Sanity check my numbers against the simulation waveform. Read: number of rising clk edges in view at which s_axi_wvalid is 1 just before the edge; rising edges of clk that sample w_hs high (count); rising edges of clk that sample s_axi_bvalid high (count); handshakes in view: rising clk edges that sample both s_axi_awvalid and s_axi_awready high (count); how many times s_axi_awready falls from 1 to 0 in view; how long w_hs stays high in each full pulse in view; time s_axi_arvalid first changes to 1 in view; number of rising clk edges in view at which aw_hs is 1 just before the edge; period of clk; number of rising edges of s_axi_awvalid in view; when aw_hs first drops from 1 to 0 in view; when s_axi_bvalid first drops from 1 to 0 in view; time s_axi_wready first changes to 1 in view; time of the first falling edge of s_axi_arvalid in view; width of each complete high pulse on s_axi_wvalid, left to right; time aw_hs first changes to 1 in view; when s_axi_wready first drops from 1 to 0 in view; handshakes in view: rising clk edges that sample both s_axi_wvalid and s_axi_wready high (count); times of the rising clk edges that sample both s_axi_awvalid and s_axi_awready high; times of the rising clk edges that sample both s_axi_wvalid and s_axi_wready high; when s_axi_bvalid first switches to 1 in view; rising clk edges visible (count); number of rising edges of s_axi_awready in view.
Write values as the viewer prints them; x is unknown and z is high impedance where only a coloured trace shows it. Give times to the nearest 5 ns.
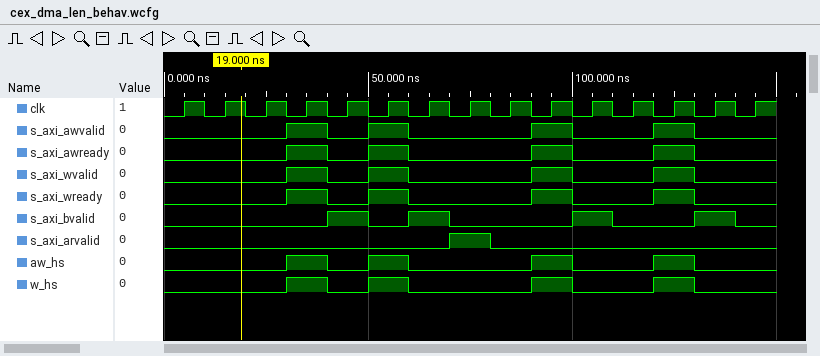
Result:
4
4
4
4
4
10 ns, 10 ns, 10 ns, 10 ns
70 ns
4
10 ns
4
40 ns
50 ns
30 ns
80 ns
10 ns, 10 ns, 10 ns, 10 ns
30 ns
40 ns
4
35 ns, 55 ns, 95 ns, 125 ns
35 ns, 55 ns, 95 ns, 125 ns
40 ns
15
4
